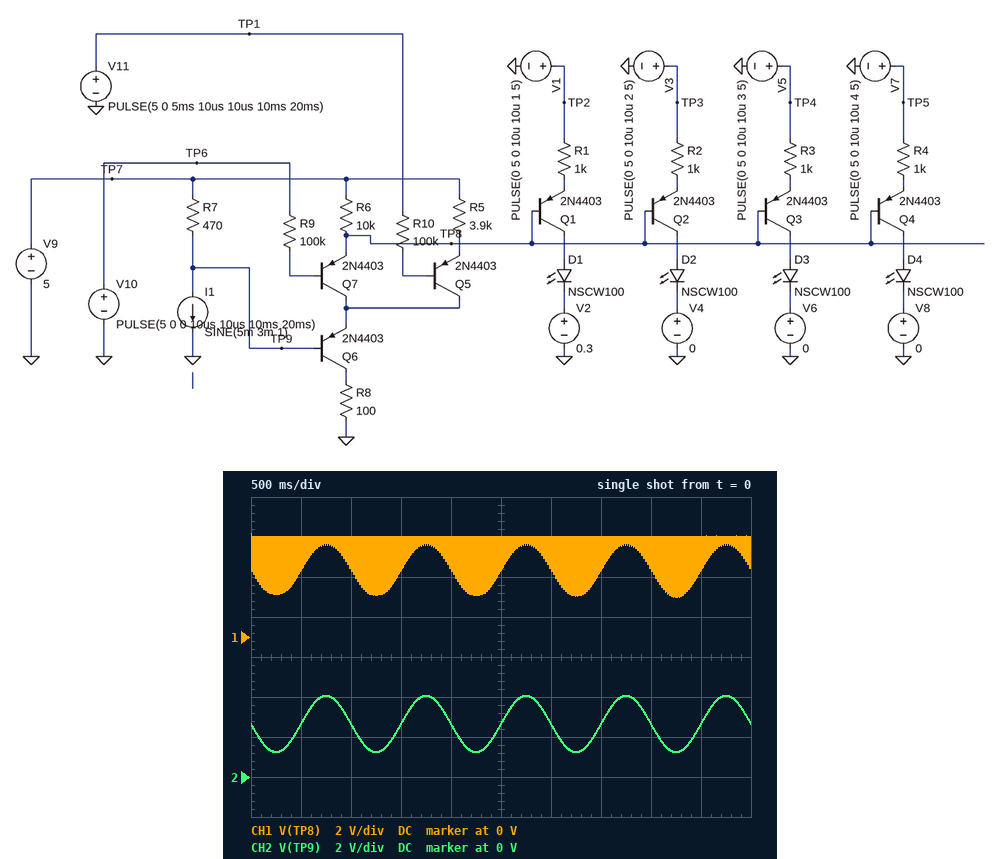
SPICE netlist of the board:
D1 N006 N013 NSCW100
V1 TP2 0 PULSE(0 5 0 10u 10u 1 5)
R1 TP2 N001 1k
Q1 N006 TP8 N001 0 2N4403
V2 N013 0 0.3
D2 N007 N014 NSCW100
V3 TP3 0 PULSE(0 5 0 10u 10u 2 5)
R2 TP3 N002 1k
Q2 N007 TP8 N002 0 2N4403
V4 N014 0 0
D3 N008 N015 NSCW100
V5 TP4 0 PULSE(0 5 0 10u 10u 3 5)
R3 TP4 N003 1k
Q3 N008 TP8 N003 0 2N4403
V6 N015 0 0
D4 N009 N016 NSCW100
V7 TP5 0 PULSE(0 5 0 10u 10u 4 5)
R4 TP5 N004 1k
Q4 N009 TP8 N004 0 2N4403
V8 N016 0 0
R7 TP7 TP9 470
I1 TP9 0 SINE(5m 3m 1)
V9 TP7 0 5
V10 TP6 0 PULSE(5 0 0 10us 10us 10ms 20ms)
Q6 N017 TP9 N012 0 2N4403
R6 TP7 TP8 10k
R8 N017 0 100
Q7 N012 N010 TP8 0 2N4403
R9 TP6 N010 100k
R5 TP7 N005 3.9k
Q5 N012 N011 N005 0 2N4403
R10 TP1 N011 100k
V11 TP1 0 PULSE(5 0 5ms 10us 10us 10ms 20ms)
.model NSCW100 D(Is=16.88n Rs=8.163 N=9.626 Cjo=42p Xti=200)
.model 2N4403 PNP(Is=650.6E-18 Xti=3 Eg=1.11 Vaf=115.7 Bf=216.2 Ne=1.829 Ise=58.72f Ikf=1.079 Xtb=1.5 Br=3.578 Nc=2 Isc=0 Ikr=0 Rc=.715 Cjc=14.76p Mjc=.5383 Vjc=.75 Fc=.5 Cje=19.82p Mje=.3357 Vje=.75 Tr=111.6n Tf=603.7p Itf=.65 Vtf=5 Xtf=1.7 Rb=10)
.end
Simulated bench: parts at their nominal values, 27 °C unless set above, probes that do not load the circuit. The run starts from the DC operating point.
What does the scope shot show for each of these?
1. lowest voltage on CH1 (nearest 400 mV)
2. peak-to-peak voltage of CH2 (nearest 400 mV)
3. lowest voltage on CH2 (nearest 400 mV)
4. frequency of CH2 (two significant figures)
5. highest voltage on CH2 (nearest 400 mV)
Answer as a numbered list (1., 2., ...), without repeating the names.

1. 2.0 V
2. 2.8 V
3. 1.2 V
4. 1.0 Hz
5. 4.0 V
